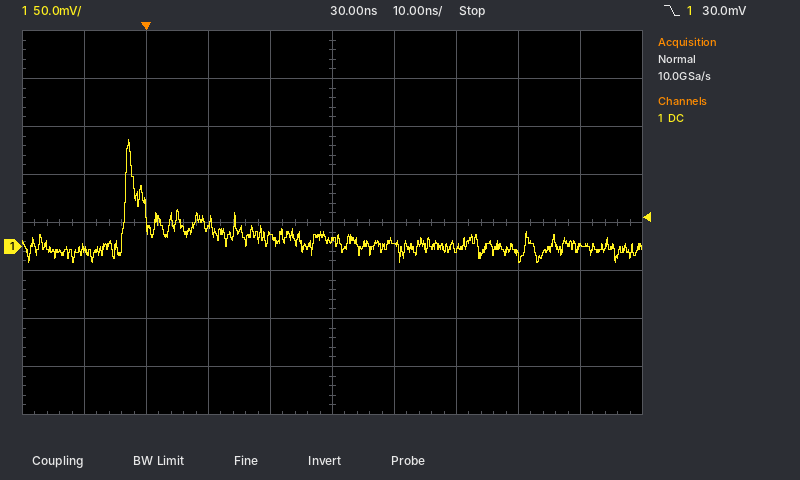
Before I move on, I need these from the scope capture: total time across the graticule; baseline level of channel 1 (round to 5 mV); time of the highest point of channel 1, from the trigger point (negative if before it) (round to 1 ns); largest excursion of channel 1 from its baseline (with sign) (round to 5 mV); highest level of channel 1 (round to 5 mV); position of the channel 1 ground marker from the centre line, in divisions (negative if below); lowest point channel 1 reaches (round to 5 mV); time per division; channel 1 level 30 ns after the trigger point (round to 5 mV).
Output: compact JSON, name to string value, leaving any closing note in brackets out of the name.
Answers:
{"total time across the graticule": "100 ns", "baseline level of channel 1": "0 mV", "time of the highest point of channel 1, from the trigger point (negative if before it)": "-3 ns", "largest excursion of channel 1 from its baseline (with sign)": "+110 mV", "highest level of channel 1": "110 mV", "position of the channel 1 ground marker from the centre line, in divisions": "-0.5 div", "lowest point channel 1 reaches": "-15 mV", "time per division": "10 ns", "channel 1 level 30 ns after the trigger point": "5 mV"}
